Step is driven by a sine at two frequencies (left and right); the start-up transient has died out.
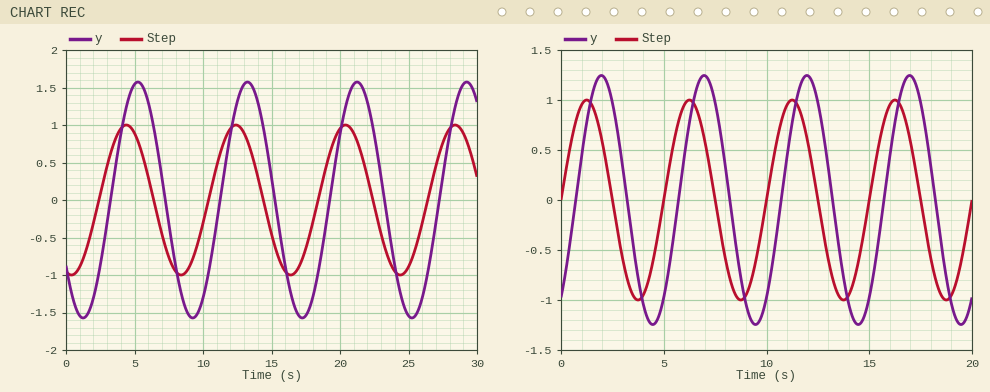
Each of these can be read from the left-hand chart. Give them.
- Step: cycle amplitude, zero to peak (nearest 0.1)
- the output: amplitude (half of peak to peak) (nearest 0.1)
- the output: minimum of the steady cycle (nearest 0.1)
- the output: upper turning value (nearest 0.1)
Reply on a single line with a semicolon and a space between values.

1.0; 1.6; -1.6; 1.6
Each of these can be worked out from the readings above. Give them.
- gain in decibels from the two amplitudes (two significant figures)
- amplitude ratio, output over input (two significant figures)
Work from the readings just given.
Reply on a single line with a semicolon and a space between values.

4.1 dB; 1.6
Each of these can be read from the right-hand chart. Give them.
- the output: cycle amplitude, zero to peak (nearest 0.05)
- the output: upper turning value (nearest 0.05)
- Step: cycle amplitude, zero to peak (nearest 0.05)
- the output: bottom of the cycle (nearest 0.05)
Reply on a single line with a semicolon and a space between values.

1.25; 1.25; 1.00; -1.25
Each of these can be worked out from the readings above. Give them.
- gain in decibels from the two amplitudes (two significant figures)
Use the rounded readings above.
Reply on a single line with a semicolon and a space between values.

1.9 dB
